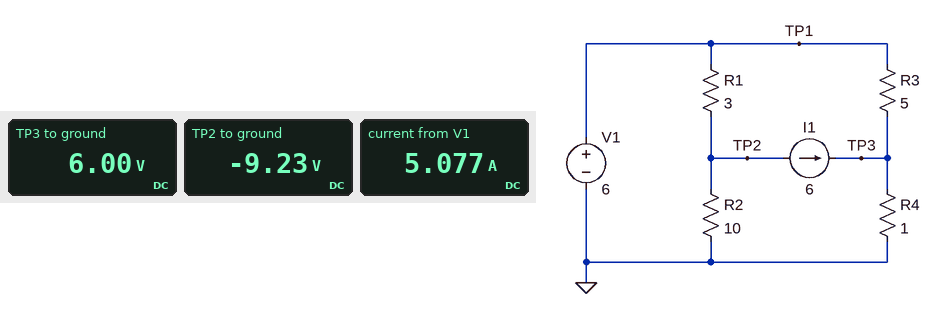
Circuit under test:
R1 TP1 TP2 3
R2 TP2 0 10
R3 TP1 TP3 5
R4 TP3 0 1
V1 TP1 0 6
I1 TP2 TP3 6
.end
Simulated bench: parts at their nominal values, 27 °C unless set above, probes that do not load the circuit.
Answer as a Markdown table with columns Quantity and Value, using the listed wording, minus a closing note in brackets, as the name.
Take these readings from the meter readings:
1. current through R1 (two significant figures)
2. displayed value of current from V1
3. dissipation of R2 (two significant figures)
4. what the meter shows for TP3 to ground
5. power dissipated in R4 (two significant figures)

| Quantity | Value |
|---|---|
| current through R1 | 5.1 A |
| displayed value of current from V1 | 5.077 A |
| dissipation of R2 | 8.5 W |
| what the meter shows for TP3 to ground | 6.00 V |
| power dissipated in R4 | 36 W |
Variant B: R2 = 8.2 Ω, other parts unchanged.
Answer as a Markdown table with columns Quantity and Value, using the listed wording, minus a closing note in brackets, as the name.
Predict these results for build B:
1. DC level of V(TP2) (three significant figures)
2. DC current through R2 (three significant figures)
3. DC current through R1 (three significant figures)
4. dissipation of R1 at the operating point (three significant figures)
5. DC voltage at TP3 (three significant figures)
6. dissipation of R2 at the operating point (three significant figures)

| Quantity | Value |
|---|---|
| DC level of V(TP2) | -8.79 V |
| DC current through R2 | 1.07 A |
| DC current through R1 | 4.93 A |
| dissipation of R1 at the operating point | 72.9 W |
| DC voltage at TP3 | 6.00 V |
| dissipation of R2 at the operating point | 9.41 W |
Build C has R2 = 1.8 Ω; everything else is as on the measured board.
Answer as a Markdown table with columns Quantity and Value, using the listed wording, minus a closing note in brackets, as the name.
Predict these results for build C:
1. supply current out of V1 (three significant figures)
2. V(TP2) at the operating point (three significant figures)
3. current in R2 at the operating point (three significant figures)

| Quantity | Value |
|---|---|
| supply current out of V1 | 3.50 A |
| V(TP2) at the operating point | -4.50 V |
| current in R2 at the operating point | 2.50 A |
